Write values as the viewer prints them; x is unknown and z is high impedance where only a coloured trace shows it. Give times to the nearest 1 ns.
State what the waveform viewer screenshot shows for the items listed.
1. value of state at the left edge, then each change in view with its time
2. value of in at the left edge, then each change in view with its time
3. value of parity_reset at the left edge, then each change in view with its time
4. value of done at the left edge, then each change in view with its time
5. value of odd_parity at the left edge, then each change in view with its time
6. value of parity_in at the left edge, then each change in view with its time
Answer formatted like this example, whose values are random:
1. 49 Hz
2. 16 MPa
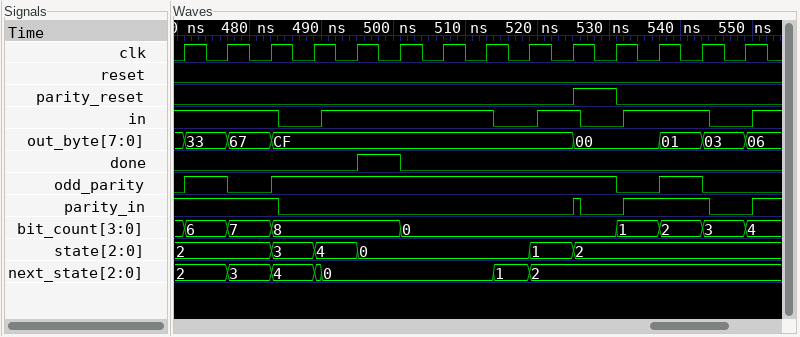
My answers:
1. 2, 3 at 483 ns, 4 at 489 ns, 0 at 495 ns, 1 at 519 ns, 2 at 525 ns
2. 1, 0 at 484 ns, 1 at 490 ns, 0 at 514 ns, 1 at 520 ns, 0 at 526 ns, 1 at 532 ns, 0 at 544 ns, 1 at 550 ns
3. 0, 1 at 525 ns, 0 at 531 ns
4. 0, 1 at 495 ns, 0 at 501 ns
5. 0, 1 at 471 ns, 0 at 477 ns, 1 at 483 ns, 0 at 531 ns, 1 at 537 ns, 0 at 543 ns
6. 1, 0 at 484 ns, 1 at 525 ns, 0 at 526 ns, 1 at 532 ns, 0 at 544 ns, 1 at 550 ns
